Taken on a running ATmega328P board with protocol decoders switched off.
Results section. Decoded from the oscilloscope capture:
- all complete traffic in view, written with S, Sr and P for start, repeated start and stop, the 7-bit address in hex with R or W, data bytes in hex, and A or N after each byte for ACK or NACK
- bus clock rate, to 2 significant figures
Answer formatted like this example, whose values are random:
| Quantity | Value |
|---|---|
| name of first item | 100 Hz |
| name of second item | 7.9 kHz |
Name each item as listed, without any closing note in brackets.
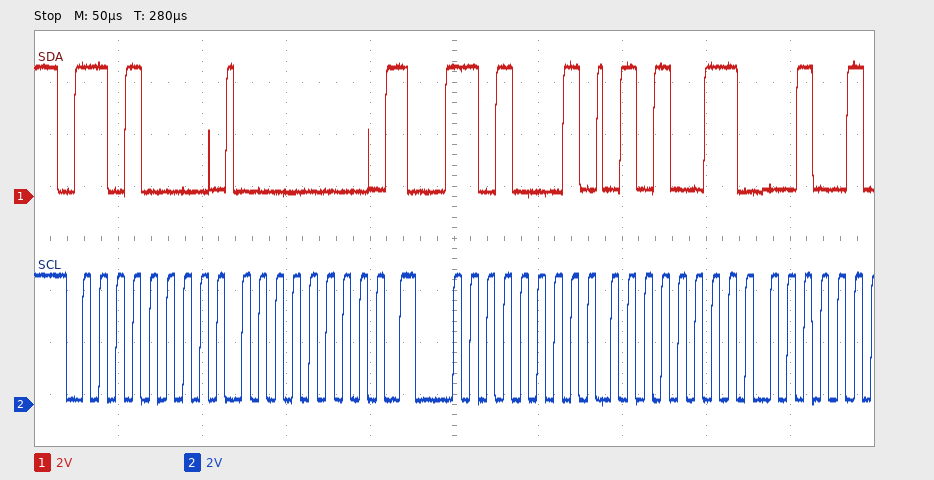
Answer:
| Quantity | Value |
|---|---|
| all complete traffic in view, written with S, Sr and P for start, repeated start and stop, the 7-bit address in hex with R or W, data bytes in hex, and A or N after each byte for ACK or NACK | S 68W A 00 A Sr 68R A 53 A |
| bus clock rate, to 2 significant figures | 100 kHz |
